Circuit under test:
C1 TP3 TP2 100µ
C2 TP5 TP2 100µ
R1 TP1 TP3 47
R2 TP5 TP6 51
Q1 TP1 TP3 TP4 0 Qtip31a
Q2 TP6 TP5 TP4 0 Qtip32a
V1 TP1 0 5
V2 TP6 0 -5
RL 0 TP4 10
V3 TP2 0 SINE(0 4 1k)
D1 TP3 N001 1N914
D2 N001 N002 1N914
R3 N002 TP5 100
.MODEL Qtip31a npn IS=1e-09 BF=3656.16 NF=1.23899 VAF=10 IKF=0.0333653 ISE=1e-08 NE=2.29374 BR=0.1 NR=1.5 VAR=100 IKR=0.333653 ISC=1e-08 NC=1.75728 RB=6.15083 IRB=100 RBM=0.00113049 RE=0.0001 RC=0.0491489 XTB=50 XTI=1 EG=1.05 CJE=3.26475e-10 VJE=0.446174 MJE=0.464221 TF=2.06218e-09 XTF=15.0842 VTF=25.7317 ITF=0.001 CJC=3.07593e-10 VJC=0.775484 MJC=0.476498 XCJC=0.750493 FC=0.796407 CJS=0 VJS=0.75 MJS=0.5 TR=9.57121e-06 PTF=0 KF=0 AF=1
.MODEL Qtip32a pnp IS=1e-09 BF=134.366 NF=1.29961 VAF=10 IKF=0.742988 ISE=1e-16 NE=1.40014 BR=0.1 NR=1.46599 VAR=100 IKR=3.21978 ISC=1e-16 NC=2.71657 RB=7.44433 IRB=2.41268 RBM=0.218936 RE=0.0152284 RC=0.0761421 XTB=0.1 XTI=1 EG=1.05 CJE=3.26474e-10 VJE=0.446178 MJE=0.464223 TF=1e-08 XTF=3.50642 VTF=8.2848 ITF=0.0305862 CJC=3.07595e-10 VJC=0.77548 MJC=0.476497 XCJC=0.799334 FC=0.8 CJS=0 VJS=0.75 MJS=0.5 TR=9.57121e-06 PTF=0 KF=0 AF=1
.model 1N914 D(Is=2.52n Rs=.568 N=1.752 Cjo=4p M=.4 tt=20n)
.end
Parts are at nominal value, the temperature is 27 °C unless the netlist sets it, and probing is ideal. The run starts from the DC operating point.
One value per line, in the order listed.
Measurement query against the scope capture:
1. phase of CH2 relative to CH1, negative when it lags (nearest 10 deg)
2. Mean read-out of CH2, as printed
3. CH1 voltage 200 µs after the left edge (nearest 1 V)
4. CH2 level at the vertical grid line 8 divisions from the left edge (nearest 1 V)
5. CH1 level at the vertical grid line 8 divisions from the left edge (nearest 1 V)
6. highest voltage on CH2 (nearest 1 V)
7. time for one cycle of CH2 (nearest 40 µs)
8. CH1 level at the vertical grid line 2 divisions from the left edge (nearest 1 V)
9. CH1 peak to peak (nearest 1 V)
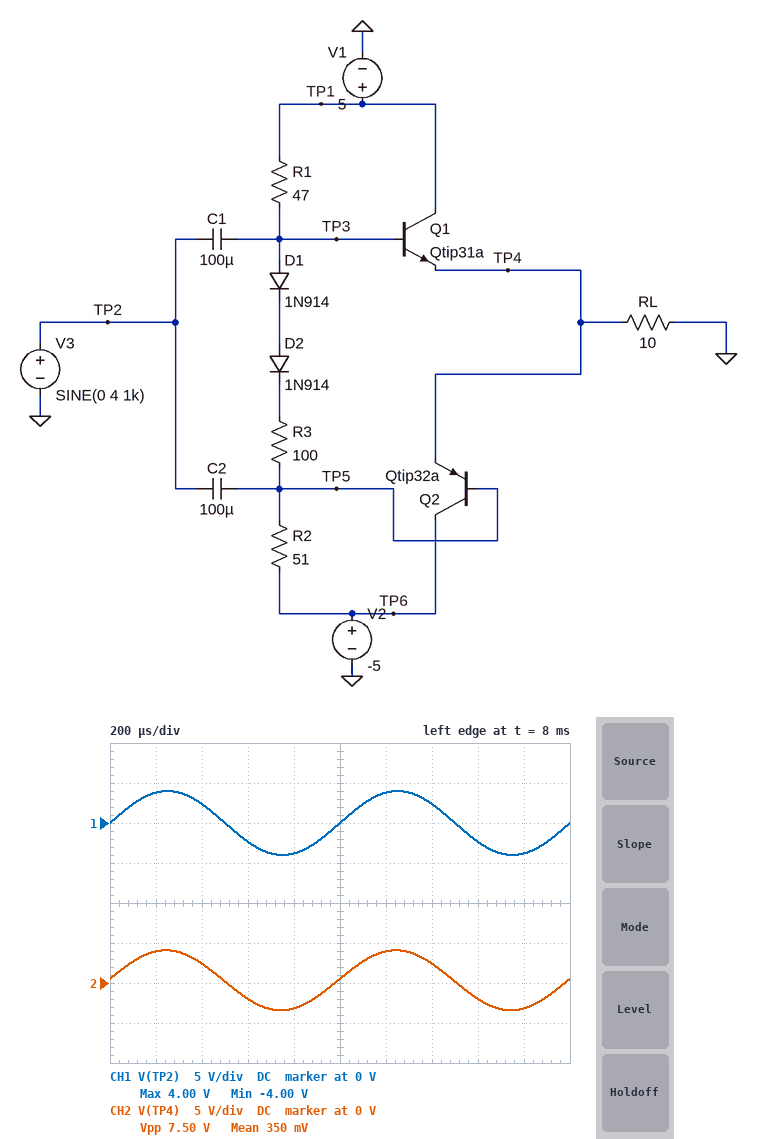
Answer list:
0 deg
350 mV
4 V
-2 V
-2 V
4 V
1.00 ms
2 V
8 V
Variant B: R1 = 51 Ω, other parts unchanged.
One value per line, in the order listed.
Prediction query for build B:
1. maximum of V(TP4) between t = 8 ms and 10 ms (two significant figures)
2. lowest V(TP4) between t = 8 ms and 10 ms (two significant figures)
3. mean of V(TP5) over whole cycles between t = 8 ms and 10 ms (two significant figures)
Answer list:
4.0 V
-3.5 V
-1.0 V
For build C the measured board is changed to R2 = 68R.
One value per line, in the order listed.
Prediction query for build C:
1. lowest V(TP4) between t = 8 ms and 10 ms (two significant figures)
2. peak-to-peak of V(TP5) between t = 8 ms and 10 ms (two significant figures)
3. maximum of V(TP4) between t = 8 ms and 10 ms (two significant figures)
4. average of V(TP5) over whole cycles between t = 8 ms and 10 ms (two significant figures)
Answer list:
-3.1 V
8.0 V
4.5 V
-500 mV
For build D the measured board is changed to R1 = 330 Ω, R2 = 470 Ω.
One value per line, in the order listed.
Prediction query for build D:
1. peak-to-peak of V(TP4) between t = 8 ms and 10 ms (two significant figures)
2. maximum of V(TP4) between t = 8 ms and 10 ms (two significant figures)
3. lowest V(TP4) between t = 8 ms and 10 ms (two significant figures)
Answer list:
7.9 V
4.7 V
-3.2 V
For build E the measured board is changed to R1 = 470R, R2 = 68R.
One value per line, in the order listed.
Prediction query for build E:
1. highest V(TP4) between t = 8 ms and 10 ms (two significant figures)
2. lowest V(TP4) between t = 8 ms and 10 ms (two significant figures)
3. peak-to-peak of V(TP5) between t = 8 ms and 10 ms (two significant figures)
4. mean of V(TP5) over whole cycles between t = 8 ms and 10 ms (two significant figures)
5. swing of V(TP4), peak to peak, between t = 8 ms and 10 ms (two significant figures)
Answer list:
2.2 V
-4.9 V
8.0 V
-2.6 V
7.1 V
